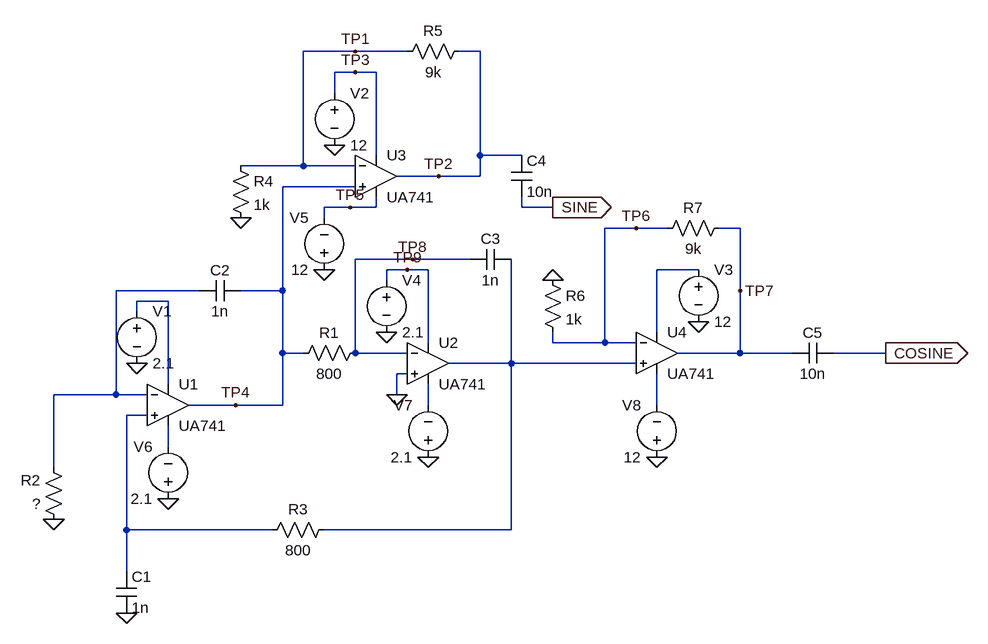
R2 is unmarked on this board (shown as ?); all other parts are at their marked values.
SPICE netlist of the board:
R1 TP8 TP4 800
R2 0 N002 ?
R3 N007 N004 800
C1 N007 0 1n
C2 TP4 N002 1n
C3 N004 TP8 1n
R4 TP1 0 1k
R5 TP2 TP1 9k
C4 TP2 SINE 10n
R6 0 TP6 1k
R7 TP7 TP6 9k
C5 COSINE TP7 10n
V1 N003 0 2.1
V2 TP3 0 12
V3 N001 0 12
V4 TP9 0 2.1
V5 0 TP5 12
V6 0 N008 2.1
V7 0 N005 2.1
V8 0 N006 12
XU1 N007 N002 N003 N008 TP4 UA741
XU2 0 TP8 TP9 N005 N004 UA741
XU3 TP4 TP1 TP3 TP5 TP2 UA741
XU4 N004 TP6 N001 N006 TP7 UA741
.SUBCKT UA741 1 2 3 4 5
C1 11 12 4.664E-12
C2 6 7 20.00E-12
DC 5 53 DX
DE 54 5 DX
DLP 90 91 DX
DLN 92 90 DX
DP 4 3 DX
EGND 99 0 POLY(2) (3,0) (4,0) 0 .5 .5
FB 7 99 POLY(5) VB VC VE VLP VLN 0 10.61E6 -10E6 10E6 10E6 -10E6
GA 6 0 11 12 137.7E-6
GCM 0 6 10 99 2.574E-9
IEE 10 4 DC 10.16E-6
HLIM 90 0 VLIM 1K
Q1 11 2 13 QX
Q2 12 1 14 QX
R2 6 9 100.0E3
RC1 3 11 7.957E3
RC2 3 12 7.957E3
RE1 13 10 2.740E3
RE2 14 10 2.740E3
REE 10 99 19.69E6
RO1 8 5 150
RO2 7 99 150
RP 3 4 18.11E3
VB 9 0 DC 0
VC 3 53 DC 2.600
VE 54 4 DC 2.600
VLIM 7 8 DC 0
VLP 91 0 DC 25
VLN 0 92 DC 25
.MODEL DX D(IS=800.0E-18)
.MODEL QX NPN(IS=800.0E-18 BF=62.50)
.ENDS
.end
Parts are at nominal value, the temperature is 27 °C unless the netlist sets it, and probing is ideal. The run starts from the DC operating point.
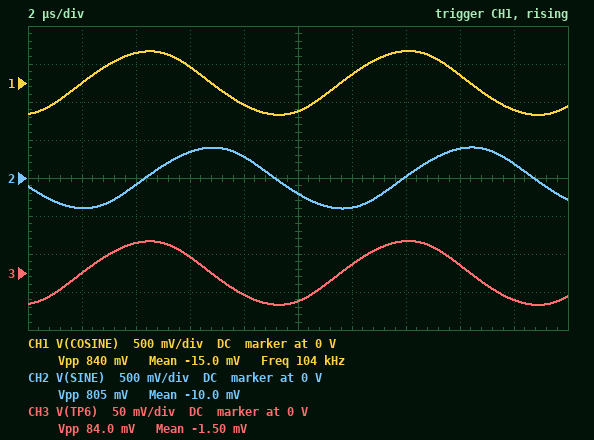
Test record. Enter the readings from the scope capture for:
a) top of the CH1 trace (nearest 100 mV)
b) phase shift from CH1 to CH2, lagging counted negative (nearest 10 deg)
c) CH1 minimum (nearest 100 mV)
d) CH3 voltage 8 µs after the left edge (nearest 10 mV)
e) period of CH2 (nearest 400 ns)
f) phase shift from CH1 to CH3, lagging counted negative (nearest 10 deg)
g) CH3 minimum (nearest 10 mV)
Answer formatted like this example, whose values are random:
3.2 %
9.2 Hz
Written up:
400 mV
-90 deg
-400 mV
-30 mV
9.6 µs
0 deg
-40 mV
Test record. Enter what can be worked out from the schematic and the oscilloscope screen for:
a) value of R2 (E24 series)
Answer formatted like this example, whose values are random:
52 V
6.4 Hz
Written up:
1 kΩ
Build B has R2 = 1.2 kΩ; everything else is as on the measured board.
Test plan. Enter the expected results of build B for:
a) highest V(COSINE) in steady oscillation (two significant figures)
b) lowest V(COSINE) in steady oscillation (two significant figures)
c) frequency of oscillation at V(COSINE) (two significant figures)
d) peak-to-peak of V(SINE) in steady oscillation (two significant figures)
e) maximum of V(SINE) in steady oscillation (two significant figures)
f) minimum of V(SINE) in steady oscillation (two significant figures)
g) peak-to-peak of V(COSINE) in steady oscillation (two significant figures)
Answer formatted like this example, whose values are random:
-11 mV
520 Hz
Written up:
280 mV
-280 mV
110 kHz
520 mV
260 mV
-260 mV
560 mV
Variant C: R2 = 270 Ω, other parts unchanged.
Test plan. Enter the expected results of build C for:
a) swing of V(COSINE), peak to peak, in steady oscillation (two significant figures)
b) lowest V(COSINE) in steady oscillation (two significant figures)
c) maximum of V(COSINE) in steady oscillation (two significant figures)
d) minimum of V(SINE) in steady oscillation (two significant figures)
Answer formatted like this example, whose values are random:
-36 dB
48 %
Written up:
1.2 V
-580 mV
580 mV
-620 mV
